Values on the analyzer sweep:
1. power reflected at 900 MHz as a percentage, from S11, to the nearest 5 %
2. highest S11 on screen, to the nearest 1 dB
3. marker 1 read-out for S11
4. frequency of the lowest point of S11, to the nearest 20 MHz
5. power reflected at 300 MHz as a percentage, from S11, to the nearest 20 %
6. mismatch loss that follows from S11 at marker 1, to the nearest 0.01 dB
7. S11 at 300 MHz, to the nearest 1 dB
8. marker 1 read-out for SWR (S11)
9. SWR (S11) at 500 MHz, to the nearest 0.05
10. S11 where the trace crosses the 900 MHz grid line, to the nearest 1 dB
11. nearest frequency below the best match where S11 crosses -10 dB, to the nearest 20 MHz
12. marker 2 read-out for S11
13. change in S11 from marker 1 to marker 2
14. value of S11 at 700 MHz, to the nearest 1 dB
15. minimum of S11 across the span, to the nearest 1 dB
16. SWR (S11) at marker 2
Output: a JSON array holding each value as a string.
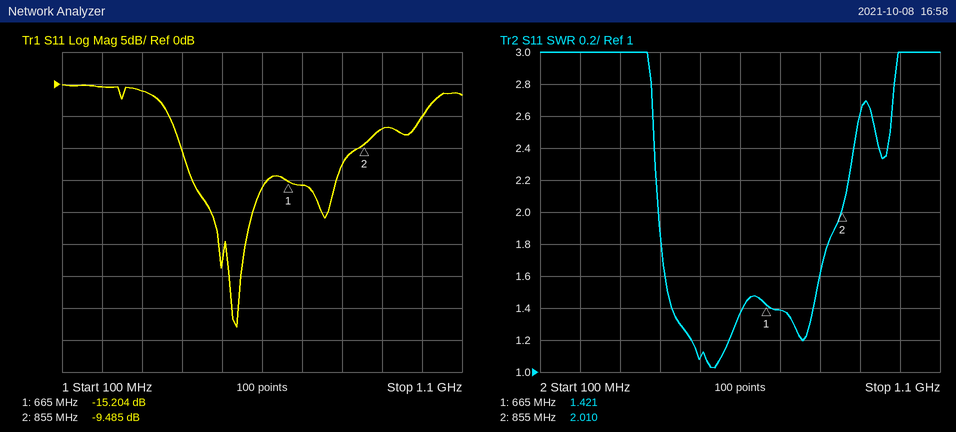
["20 %", "0 dB", "-15.204 dB", "540 MHz", "80 %", "0.13 dB", "-1 dB", "1.421", "1.10", "-7 dB", "400 MHz", "-9.485 dB", "5.719 dB", "-16 dB", "-38 dB", "2.010"]
